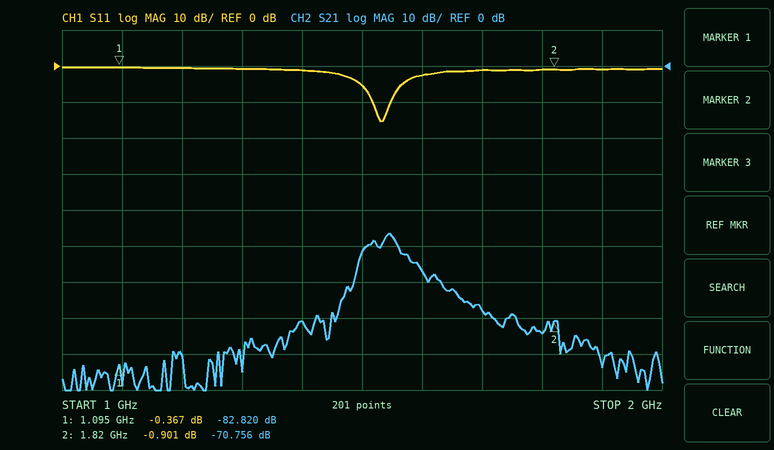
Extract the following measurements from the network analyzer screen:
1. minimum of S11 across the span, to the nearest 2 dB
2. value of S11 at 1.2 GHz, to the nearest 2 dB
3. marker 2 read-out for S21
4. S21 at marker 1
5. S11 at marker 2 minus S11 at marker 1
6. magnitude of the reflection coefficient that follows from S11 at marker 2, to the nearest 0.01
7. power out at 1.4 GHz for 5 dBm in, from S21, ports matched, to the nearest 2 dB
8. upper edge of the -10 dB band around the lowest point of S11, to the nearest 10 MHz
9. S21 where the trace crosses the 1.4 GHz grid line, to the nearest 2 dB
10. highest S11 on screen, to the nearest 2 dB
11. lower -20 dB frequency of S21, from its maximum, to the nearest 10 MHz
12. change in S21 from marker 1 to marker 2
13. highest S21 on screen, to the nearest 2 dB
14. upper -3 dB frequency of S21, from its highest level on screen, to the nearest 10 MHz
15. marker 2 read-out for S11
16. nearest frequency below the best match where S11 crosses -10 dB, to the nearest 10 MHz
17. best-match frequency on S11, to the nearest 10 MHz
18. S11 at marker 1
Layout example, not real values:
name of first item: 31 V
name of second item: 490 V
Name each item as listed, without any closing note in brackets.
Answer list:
minimum of S11 across the span, to the nearest 2 dB: -16 dB
value of S11 at 1.2 GHz, to the nearest 2 dB: 0 dB
marker 2 read-out for S21: -70.756 dB
S21 at marker 1: -82.820 dB
S11 at marker 2 minus S11 at marker 1: -0.534 dB
magnitude of the reflection coefficient that follows from S11 at marker 2, to the nearest 0.01: 0.90
power out at 1.4 GHz for 5 dBm in, from S21, ports matched, to the nearest 2 dB: -66 dBm
upper edge of the -10 dB band around the lowest point of S11, to the nearest 10 MHz: 1.55 GHz
S21 where the trace crosses the 1.4 GHz grid line, to the nearest 2 dB: -70 dB
highest S11 on screen, to the nearest 2 dB: 0 dB
lower -20 dB frequency of S21, from its maximum, to the nearest 10 MHz: 1.46 GHz
change in S21 from marker 1 to marker 2: 12.064 dB
highest S21 on screen, to the nearest 2 dB: -46 dB
upper -3 dB frequency of S21, from its highest level on screen, to the nearest 10 MHz: 1.56 GHz
marker 2 read-out for S11: -0.901 dB
nearest frequency below the best match where S11 crosses -10 dB, to the nearest 10 MHz: 1.52 GHz
best-match frequency on S11, to the nearest 10 MHz: 1.53 GHz
S11 at marker 1: -0.367 dB
